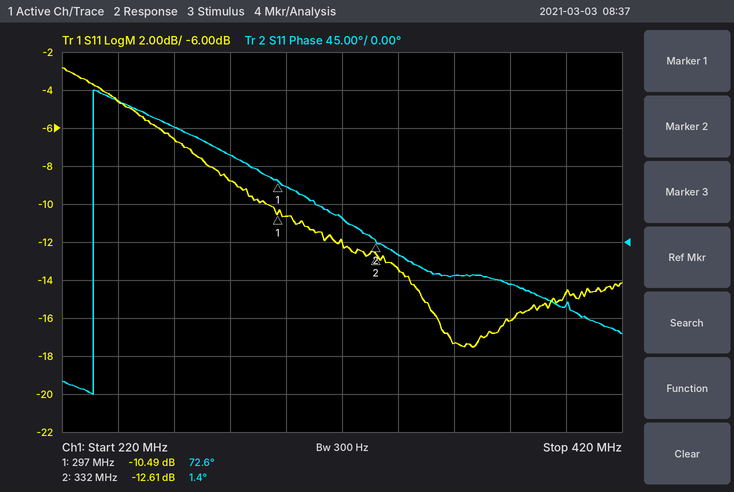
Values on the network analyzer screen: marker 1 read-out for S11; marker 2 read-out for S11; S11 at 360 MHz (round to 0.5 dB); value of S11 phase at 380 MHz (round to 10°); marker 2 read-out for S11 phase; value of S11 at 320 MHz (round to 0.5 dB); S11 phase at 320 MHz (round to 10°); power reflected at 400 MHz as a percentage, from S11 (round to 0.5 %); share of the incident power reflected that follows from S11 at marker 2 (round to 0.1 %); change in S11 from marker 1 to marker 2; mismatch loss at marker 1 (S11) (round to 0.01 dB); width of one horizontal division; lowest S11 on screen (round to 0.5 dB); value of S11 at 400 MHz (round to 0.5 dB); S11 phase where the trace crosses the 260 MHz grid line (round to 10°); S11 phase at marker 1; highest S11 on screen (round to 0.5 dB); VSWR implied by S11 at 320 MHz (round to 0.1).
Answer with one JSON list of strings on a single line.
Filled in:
["-10.49 dB", "-12.61 dB", "-17.5 dB", "-50°", "1.4°", "-12.0 dB", "30°", "3.5 %", "5.5 %", "-2.12 dB", "0.41 dB", "20 MHz", "-17.5 dB", "-14.5 dB", "140°", "72.6°", "-3.0 dB", "1.7"]
